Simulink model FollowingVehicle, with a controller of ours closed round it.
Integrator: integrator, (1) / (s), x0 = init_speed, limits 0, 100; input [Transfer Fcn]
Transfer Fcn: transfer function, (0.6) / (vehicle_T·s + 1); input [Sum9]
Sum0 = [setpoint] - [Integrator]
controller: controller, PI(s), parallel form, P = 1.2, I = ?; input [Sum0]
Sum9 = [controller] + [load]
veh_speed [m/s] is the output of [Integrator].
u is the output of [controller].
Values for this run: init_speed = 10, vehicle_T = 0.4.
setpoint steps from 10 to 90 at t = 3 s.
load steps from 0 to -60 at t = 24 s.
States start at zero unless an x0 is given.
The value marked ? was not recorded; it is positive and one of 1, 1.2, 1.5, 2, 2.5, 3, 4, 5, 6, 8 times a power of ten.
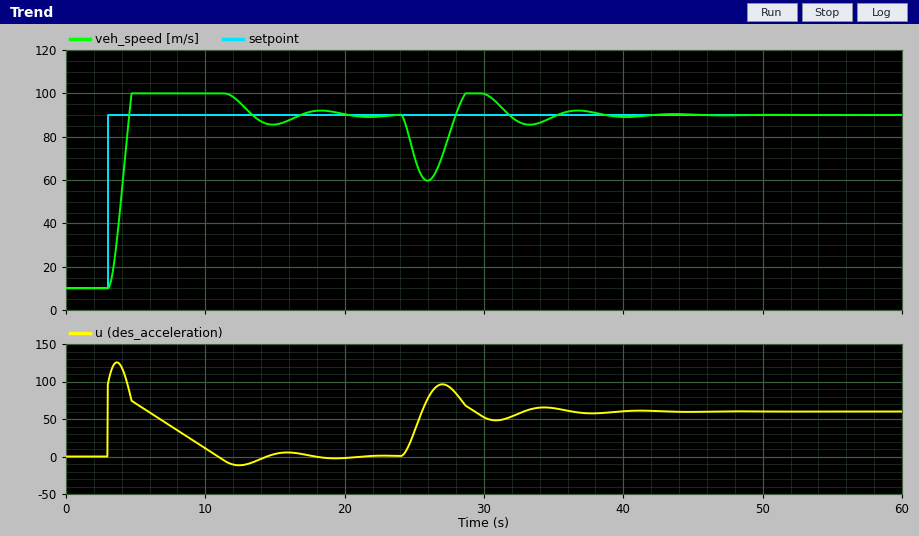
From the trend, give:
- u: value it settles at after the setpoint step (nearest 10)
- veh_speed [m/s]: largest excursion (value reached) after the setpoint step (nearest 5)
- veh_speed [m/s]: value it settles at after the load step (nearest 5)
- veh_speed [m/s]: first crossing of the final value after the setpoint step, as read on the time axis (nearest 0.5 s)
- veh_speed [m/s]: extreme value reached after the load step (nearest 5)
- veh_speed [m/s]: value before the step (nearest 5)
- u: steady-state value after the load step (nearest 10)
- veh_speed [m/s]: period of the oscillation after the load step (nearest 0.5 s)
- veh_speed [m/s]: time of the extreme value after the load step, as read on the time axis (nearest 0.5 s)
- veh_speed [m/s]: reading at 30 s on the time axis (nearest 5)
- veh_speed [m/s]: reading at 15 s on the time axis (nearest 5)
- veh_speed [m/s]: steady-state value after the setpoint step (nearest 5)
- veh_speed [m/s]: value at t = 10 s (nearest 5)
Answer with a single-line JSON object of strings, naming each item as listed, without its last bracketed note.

{"u: value it settles at after the setpoint step": "0", "veh_speed [m/s]: largest excursion (value reached) after the setpoint step": "100", "veh_speed [m/s]: value it settles at after the load step": "90", "veh_speed [m/s]: first crossing of the final value after the setpoint step, as read on the time axis": "4.5 s", "veh_speed [m/s]: extreme value reached after the load step": "60", "veh_speed [m/s]: value before the step": "10", "u: steady-state value after the load step": "60", "veh_speed [m/s]: period of the oscillation after the load step": "7.5 s", "veh_speed [m/s]: time of the extreme value after the load step, as read on the time axis": "26.0 s", "veh_speed [m/s]: reading at 30 s on the time axis": "100", "veh_speed [m/s]: reading at 15 s on the time axis": "85", "veh_speed [m/s]: steady-state value after the setpoint step": "90", "veh_speed [m/s]: value at t = 10 s": "100"}
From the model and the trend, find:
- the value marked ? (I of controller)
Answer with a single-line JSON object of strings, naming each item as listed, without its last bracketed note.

{"the value marked ?": "1.2"}
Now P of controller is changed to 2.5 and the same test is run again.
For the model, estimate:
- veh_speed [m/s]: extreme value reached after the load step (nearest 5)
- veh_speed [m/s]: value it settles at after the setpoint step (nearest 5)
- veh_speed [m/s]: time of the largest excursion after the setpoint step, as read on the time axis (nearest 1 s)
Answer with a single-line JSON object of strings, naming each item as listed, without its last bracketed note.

{"veh_speed [m/s]: extreme value reached after the load step": "70", "veh_speed [m/s]: value it settles at after the setpoint step": "90", "veh_speed [m/s]: time of the largest excursion after the setpoint step, as read on the time axis": "4 s"}
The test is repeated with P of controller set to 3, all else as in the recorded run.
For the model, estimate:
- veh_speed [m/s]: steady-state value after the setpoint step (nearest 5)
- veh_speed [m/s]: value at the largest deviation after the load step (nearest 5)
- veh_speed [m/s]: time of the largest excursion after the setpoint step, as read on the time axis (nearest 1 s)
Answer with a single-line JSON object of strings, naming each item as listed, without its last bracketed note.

{"veh_speed [m/s]: steady-state value after the setpoint step": "90", "veh_speed [m/s]: value at the largest deviation after the load step": "70", "veh_speed [m/s]: time of the largest excursion after the setpoint step, as read on the time axis": "4 s"}
